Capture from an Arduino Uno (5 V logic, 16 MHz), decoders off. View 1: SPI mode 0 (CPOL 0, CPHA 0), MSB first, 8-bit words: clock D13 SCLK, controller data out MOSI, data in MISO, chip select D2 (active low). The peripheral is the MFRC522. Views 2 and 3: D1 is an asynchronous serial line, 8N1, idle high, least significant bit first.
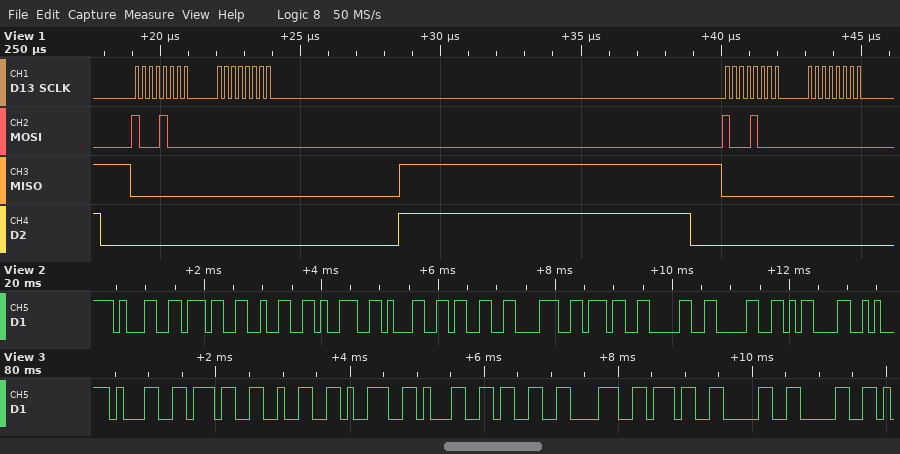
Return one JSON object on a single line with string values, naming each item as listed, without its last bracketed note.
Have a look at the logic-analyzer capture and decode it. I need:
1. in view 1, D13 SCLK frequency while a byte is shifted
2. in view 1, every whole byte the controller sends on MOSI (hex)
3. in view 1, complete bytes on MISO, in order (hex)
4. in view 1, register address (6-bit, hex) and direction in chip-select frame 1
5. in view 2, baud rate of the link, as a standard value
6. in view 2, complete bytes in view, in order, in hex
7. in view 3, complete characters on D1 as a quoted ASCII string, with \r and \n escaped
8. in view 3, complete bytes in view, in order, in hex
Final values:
{"in view 1, D13 SCLK frequency while a byte is shifted": "4 MHz", "in view 1, every whole byte the controller sends on MOSI": "88 00 88 00", "in view 1, complete bytes on MISO, in order": "00 00 00 00", "in view 1, register address (6-bit, hex) and direction in chip-select frame 1": "0x04 read", "in view 2, baud rate of the link, as a standard value": "9600 baud", "in view 2, complete bytes in view, in order, in hex": "0x31 0x37 0x32 0x39 0x31 0x33 0x38 0x37 0x30 0x30 0x0D", "in view 3, complete characters on D1 as a quoted ASCII string, with \\r and \\n escaped": "\"1729138700\"", "in view 3, complete bytes in view, in order, in hex": "31 37 32 39 31 33 38 37 30 30"}
